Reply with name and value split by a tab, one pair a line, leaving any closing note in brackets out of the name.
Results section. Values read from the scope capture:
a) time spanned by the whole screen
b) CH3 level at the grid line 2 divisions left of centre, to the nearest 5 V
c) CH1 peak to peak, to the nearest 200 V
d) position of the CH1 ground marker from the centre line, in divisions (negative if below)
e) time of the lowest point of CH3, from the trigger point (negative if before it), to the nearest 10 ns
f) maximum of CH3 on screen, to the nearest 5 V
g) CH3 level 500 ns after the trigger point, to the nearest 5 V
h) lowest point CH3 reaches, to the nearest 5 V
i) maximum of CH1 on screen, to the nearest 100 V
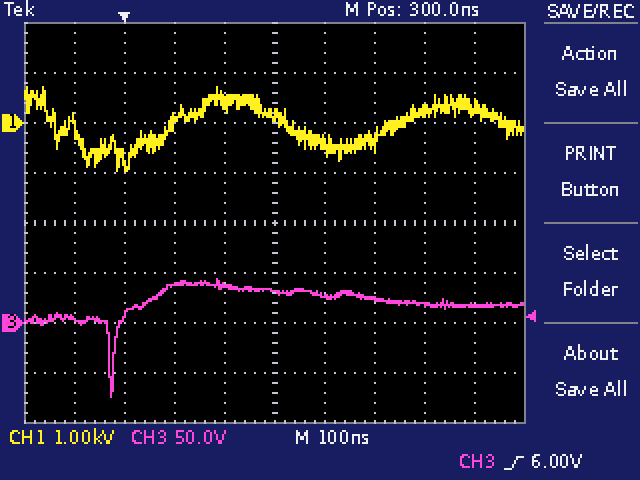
time spanned by the whole screen	1 µs
CH3 level at the grid line 2 divisions left of centre, to the nearest 5 V	40 V
CH1 peak to peak, to the nearest 200 V	1.6 kV
position of the CH1 ground marker from the centre line, in divisions	+2.0 div
time of the lowest point of CH3, from the trigger point (negative if before it), to the nearest 10 ns	-30 ns
maximum of CH3 on screen, to the nearest 5 V	45 V
CH3 level 500 ns after the trigger point, to the nearest 5 V	25 V
lowest point CH3 reaches, to the nearest 5 V	-75 V
maximum of CH1 on screen, to the nearest 100 V	700 V
